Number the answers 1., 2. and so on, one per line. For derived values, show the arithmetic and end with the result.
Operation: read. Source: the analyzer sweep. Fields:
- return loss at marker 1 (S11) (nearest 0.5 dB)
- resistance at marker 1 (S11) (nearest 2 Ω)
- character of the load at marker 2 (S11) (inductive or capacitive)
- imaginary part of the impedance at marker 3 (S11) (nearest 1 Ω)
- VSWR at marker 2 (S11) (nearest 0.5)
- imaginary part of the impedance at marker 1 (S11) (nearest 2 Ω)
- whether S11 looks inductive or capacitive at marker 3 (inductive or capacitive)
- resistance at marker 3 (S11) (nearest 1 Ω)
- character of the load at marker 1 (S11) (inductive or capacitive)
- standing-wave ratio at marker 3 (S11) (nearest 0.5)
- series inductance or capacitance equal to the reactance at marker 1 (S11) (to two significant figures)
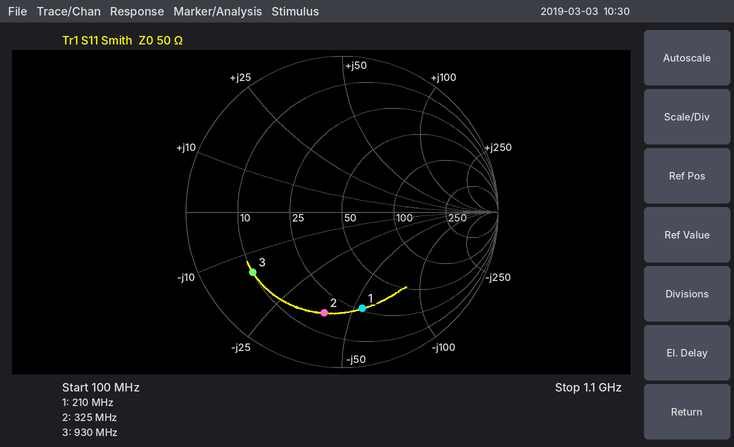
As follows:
1. 4.0 dB
2. 26 Ω
3. capacitive
4. -15 Ω
5. 5.0
6. -54 Ω
7. capacitive
8. 10 Ω
9. capacitive
10. 5.5
11. C = 1/(2π × 210 MHz × 54 Ω) ≈ 14 pF
